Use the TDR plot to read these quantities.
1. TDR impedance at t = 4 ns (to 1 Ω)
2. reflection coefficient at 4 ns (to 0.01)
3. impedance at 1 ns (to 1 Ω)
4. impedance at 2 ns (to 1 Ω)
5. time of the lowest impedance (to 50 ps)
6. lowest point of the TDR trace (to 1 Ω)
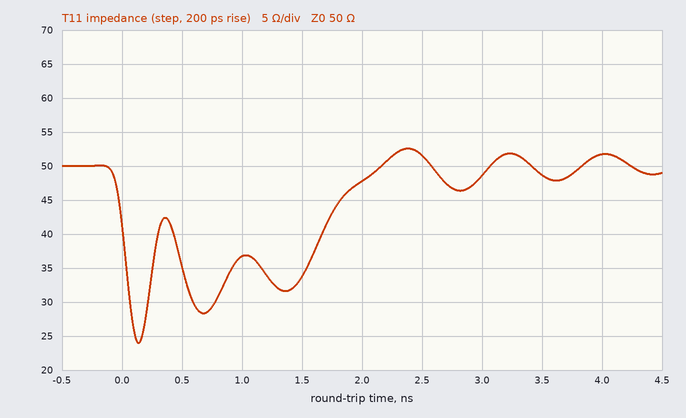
52 Ω
+0.02
37 Ω
48 Ω
150 ps
24 Ω
